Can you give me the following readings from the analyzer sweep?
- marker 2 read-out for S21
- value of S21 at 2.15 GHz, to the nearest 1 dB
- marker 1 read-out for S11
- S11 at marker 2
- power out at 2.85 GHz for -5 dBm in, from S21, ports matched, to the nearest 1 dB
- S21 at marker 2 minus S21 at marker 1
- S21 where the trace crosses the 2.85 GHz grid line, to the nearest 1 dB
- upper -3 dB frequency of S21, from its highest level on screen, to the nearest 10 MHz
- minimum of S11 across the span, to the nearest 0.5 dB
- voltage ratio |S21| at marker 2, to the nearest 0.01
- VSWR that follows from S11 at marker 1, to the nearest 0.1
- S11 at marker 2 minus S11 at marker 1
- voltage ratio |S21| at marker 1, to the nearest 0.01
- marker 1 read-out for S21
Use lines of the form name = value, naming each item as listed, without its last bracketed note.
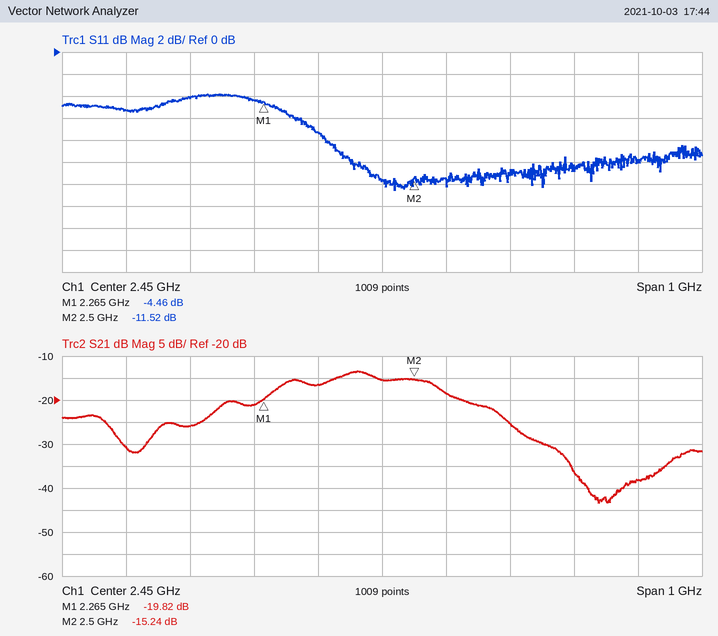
marker 2 read-out for S21 = -15.24 dB
value of S21 at 2.15 GHz, to the nearest 1 dB = -26 dB
marker 1 read-out for S11 = -4.46 dB
S11 at marker 2 = -11.52 dB
power out at 2.85 GHz for -5 dBm in, from S21, ports matched, to the nearest 1 dB = -43 dBm
S21 at marker 2 minus S21 at marker 1 = 4.58 dB
S21 where the trace crosses the 2.85 GHz grid line, to the nearest 1 dB = -38 dB
upper -3 dB frequency of S21, from its highest level on screen, to the nearest 10 MHz = 2.53 GHz
minimum of S11 across the span, to the nearest 0.5 dB = -12.5 dB
voltage ratio |S21| at marker 2, to the nearest 0.01 = 0.17
VSWR that follows from S11 at marker 1, to the nearest 0.1 = 4.0
S11 at marker 2 minus S11 at marker 1 = -7.06 dB
voltage ratio |S21| at marker 1, to the nearest 0.01 = 0.10
marker 1 read-out for S21 = -19.82 dB
